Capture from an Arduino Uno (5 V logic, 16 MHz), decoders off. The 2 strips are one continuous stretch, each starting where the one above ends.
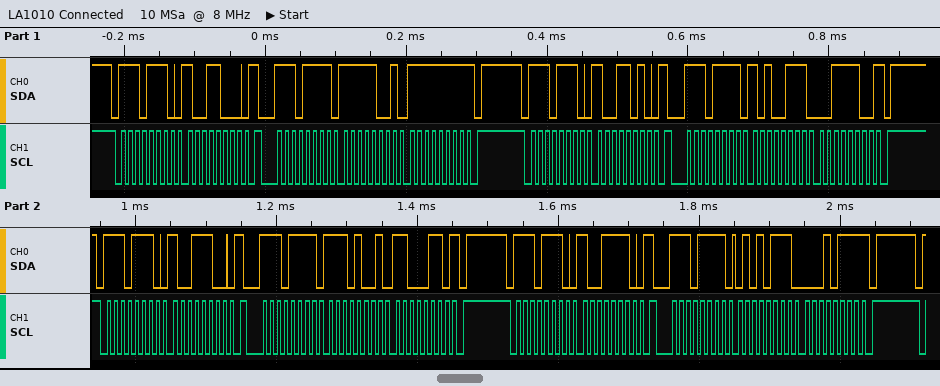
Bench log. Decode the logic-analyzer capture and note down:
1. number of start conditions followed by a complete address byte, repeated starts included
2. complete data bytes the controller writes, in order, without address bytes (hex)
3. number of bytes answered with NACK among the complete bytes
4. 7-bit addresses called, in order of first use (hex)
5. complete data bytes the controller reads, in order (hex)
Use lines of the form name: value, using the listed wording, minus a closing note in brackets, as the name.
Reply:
number of start conditions followed by a complete address byte, repeated starts included: 8
complete data bytes the controller writes, in order, without address bytes: 98 9A 9C 9E
number of bytes answered with NACK among the complete bytes: 4
7-bit addresses called, in order of first use: 0x77
complete data bytes the controller reads, in order: F9 FF A7 3C E9 C6 57 17
